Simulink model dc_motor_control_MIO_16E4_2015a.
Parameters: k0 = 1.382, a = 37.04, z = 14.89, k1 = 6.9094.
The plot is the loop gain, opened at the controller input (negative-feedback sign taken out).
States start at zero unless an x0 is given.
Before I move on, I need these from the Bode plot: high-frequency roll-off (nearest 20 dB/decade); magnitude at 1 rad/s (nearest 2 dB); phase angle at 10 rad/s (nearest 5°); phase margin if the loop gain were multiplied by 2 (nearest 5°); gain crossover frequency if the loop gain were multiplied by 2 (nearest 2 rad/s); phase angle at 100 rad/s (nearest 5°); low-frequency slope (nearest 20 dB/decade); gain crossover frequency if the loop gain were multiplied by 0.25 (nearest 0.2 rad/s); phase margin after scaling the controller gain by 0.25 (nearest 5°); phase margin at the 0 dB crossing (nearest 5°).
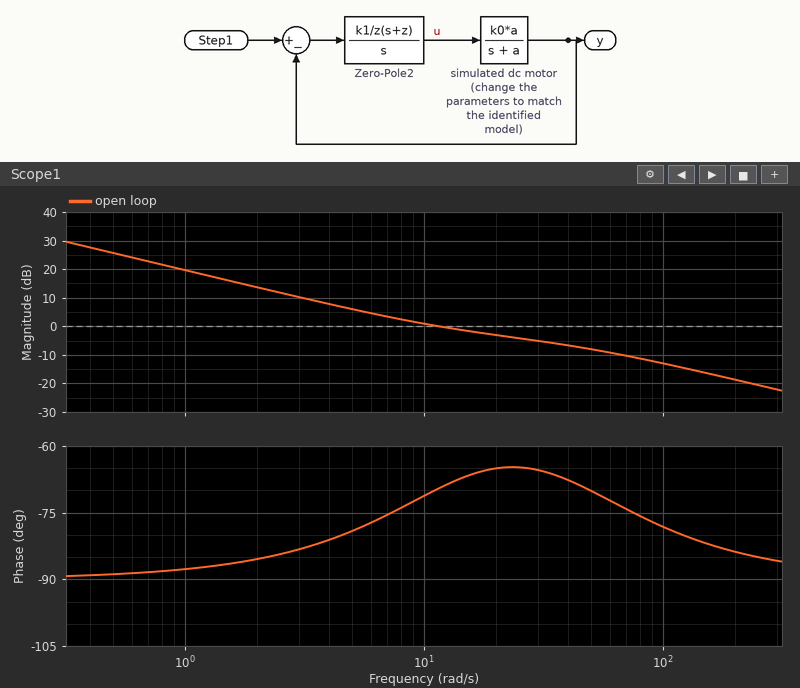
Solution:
-20 dB/decade
20 dB
-70°
115°
36 rad/s
-80°
-20 dB/decade
2.4 rad/s
95°
110°
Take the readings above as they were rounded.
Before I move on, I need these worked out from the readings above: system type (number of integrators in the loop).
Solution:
1
